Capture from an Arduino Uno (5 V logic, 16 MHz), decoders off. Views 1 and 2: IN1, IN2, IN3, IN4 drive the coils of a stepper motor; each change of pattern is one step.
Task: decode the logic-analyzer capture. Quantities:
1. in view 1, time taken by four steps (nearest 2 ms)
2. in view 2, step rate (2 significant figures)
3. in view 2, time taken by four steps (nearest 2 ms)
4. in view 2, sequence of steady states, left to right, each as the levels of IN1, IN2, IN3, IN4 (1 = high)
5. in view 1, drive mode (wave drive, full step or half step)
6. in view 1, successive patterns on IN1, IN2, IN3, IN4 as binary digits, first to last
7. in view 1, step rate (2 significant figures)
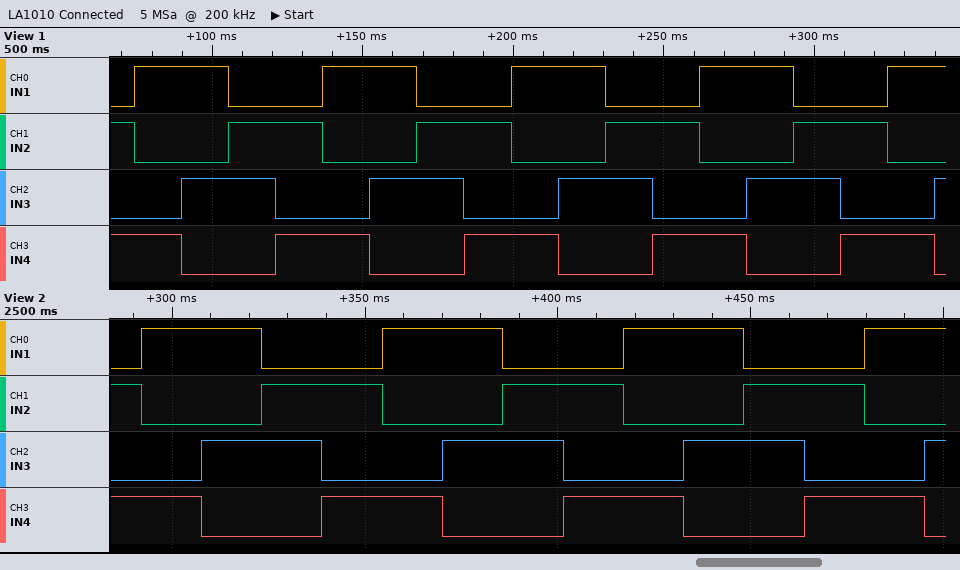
62 ms
64 steps/s
62 ms
0101 1001 1010 0110 0101 1001 1010 0110 0101 1001 1010 0110 0101 1001 1010
full step
0101 1001 1010 0110 0101 1001 1010 0110 0101 1001 1010 0110 0101 1001 1010 0110 0101 1001 1010
64 steps/s
